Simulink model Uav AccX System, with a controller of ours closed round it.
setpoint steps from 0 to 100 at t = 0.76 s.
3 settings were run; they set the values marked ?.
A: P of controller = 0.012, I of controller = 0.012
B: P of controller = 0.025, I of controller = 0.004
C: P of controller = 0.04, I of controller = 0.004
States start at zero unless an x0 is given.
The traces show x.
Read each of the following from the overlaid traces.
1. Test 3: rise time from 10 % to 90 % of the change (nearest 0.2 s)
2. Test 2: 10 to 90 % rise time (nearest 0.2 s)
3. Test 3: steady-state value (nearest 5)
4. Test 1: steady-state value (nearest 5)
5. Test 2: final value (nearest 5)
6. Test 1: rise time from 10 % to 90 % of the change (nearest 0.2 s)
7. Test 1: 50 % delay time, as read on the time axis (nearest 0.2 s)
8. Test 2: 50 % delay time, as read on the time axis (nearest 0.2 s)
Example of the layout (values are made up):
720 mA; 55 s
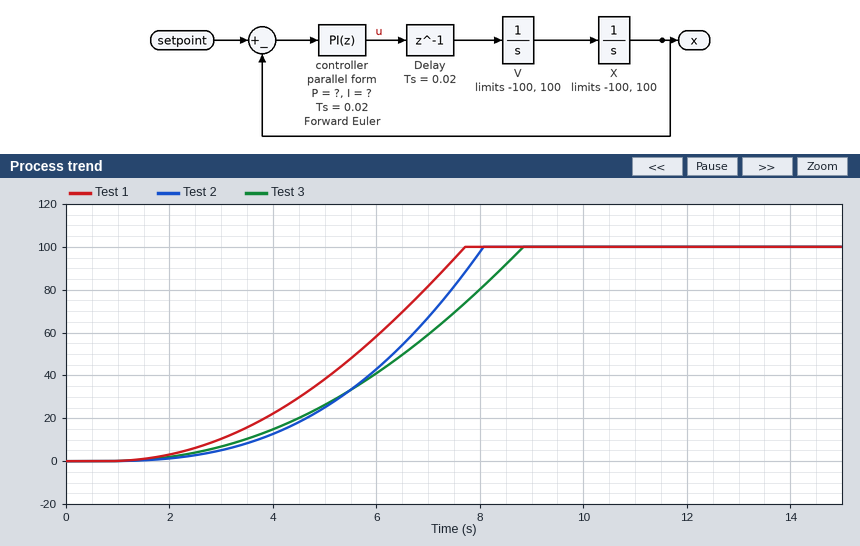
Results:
5.0 s; 4.0 s; 100; 100; 100; 4.4 s; 5.6 s; 6.4 s
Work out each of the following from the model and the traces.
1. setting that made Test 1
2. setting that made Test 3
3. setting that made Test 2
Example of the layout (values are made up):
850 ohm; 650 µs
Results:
C; B; A
